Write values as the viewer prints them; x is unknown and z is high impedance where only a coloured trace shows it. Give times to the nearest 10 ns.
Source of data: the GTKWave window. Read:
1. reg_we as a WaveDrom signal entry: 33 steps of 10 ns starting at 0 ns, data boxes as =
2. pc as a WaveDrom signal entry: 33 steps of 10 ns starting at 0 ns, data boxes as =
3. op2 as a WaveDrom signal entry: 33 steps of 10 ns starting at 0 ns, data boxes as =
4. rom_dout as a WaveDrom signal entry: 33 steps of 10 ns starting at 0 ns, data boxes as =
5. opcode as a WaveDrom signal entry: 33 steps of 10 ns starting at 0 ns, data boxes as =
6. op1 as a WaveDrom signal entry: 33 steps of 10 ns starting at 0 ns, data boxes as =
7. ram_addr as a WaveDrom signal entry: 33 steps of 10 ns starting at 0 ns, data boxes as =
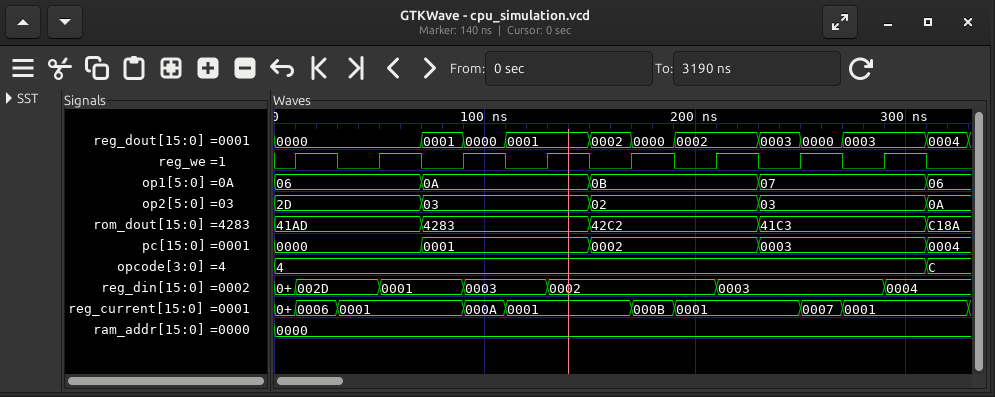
{name: 'reg_we', wave: '01.0.1.0.1.0.1.0.1.0.1.0.1.0.1.0.'}
{name: 'pc', wave: '=......=.......=.......=.......=.', data: '0000 0001 0002 0003 0004'}
{name: 'op2', wave: '=......=.......=.......=.......=.', data: '2D 03 02 03 0A'}
{name: 'rom_dout', wave: '=......=.......=.......=.......=.', data: '41AD 4283 42C2 41C3 C18A'}
{name: 'opcode', wave: '=..............................=.', data: '4 C'}
{name: 'op1', wave: '=......=.......=.......=.......=.', data: '06 0A 0B 07 06'}
{name: 'ram_addr', wave: '=................................', data: '0000'}
